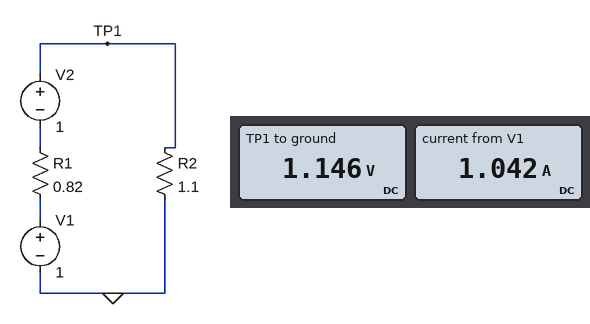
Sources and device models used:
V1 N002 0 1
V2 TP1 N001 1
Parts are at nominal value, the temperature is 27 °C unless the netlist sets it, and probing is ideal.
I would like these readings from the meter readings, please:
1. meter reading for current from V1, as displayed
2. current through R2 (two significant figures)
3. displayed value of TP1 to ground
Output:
1.042 A
1.0 A
1.146 V
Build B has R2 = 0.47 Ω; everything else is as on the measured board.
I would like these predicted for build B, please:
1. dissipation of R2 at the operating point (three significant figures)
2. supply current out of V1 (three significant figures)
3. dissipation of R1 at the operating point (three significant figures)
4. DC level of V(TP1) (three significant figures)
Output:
1.13 W
1.55 A
1.97 W
729 mV
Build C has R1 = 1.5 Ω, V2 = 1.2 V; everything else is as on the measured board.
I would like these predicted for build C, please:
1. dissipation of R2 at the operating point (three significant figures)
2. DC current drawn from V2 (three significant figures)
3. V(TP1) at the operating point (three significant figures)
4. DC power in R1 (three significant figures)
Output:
788 mW
846 mA
931 mV
1.07 W
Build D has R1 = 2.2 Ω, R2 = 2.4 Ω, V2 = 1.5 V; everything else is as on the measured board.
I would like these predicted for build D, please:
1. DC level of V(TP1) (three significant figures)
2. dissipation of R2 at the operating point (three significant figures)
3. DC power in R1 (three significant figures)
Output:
1.30 V
709 mW
650 mW
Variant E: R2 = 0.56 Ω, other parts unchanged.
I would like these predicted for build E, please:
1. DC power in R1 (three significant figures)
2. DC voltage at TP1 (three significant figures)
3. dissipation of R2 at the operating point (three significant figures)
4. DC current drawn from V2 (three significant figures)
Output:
1.72 W
812 mV
1.18 W
1.45 A
